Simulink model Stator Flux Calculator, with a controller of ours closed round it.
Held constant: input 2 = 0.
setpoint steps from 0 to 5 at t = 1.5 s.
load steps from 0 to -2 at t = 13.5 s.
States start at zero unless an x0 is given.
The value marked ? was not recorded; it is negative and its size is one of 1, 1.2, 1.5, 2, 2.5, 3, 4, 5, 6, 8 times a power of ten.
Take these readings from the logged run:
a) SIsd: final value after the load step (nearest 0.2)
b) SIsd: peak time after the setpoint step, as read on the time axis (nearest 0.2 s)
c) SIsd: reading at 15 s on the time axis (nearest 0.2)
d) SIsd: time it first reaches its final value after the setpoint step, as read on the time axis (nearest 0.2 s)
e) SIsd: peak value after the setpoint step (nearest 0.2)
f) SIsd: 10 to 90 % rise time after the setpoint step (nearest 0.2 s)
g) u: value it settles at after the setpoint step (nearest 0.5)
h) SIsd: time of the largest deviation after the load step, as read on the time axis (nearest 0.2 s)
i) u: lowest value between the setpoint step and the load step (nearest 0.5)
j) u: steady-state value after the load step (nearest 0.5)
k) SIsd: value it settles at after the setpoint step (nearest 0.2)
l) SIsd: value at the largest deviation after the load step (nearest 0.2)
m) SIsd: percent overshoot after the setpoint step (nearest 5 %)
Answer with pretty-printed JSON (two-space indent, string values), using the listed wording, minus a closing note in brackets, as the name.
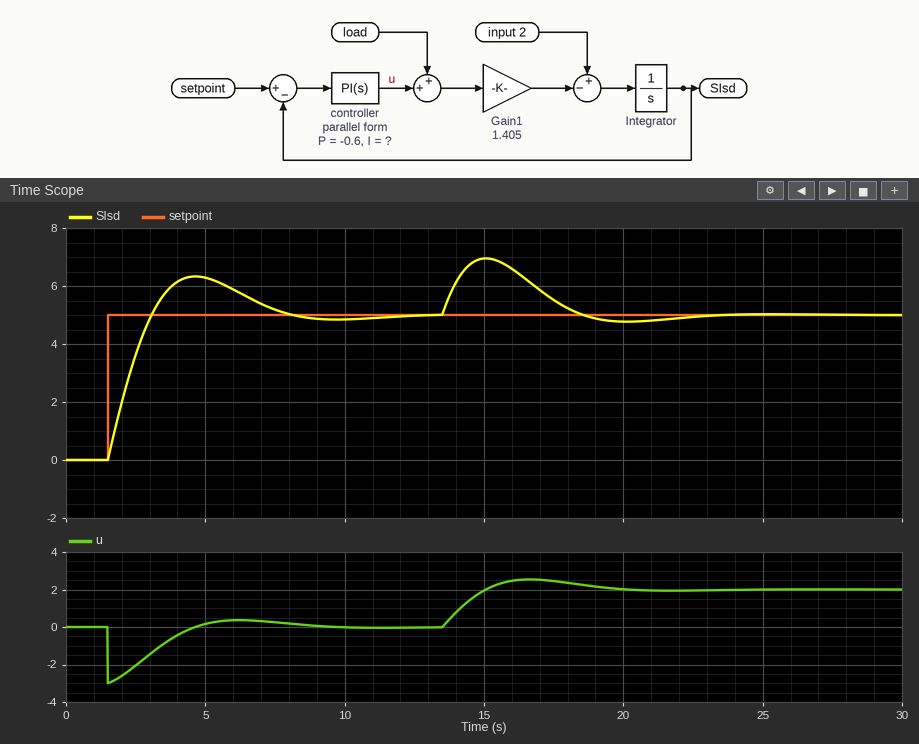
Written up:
{
  "SIsd: final value after the load step": "5.0",
  "SIsd: peak time after the setpoint step, as read on the time axis": "4.6 s",
  "SIsd: reading at 15 s on the time axis": "7.0",
  "SIsd: time it first reaches its final value after the setpoint step, as read on the time axis": "3.0 s",
  "SIsd: peak value after the setpoint step": "6.4",
  "SIsd: 10 to 90 % rise time after the setpoint step": "1.2 s",
  "u: value it settles at after the setpoint step": "0.0",
  "SIsd: time of the largest deviation after the load step, as read on the time axis": "15.0 s",
  "u: lowest value between the setpoint step and the load step": "-3.0",
  "u: steady-state value after the load step": "2.0",
  "SIsd: value it settles at after the setpoint step": "5.0",
  "SIsd: value at the largest deviation after the load step": "7.0",
  "SIsd: percent overshoot after the setpoint step": "25 %"
}
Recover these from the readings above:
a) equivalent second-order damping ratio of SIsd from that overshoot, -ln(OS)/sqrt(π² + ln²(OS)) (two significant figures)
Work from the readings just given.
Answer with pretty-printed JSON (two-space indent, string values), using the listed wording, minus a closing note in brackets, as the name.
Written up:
{
  "equivalent second-order damping ratio of SIsd from that overshoot, -ln(OS)/sqrt(π² + ln²(OS))": "0.40"
}
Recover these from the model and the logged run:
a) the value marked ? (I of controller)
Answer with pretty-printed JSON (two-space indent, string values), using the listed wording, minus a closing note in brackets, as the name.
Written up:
{
  "the value marked ?": "-0.4"
}
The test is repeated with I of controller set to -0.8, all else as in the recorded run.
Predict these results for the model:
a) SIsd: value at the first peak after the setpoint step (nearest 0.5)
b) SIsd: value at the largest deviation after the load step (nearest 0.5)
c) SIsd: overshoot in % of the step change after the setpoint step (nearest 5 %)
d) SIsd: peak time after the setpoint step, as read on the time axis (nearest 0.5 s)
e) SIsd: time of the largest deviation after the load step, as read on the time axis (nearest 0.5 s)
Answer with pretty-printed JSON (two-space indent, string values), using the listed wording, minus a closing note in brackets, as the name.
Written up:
{
  "SIsd: value at the first peak after the setpoint step": "7.0",
  "SIsd: value at the largest deviation after the load step": "6.5",
  "SIsd: overshoot in % of the step change after the setpoint step": "35 %",
  "SIsd: peak time after the setpoint step, as read on the time axis": "4.0 s",
  "SIsd: time of the largest deviation after the load step, as read on the time axis": "14.5 s"
}
